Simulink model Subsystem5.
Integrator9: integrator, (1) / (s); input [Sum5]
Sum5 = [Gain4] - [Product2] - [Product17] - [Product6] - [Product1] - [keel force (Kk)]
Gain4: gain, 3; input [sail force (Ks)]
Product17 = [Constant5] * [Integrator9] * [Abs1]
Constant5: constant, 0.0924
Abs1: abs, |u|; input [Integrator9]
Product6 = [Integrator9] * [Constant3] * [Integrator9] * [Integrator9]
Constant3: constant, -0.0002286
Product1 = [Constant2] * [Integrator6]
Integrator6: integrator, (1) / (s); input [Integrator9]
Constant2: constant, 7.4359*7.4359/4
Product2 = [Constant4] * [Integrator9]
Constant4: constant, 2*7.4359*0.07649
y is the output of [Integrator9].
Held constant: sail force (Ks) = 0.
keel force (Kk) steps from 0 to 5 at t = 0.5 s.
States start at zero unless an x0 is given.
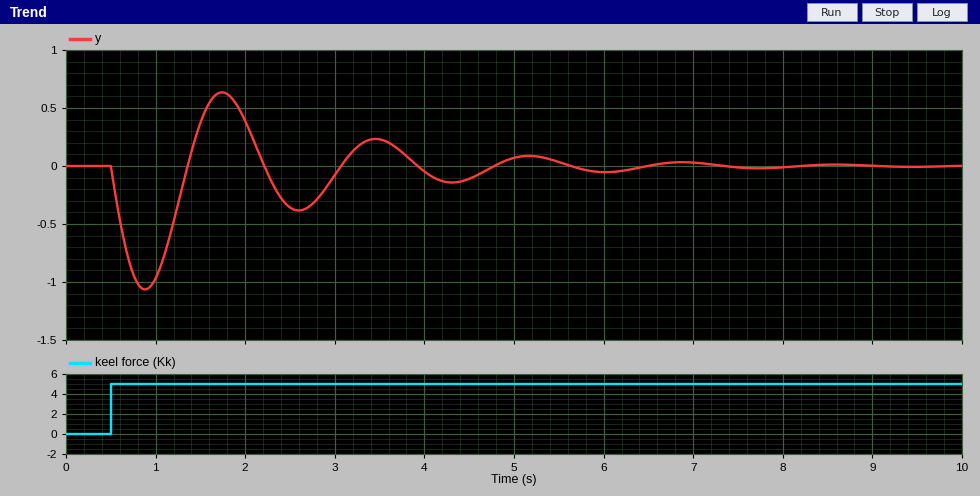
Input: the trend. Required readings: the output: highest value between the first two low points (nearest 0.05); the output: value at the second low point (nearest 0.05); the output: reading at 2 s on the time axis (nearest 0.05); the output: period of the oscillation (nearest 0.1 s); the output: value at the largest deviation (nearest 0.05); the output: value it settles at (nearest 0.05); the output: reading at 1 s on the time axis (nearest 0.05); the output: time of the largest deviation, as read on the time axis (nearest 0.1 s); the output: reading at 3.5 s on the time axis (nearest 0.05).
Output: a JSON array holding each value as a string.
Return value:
["0.65", "-0.40", "0.40", "1.7 s", "-1.05", "0.00", "-0.95", "0.9 s", "0.25"]
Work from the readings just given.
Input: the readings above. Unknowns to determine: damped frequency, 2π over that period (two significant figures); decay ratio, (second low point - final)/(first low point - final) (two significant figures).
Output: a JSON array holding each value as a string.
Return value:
["3.7 rad/s", "0.38"]
